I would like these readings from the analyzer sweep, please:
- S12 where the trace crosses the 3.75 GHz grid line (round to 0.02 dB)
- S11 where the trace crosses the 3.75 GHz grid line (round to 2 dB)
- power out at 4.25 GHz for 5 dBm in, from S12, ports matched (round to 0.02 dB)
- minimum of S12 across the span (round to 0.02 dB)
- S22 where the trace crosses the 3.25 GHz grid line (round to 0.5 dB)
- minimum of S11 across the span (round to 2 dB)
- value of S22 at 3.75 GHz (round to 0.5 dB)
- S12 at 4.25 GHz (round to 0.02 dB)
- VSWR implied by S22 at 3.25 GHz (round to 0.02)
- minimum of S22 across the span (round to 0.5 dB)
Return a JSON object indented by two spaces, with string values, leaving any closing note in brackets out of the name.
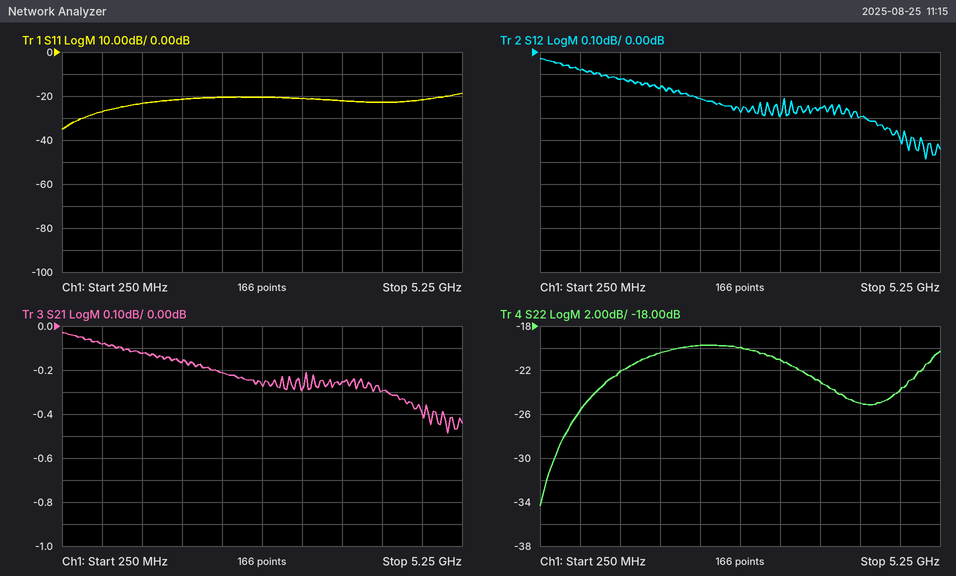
{
  "S12 where the trace crosses the 3.75 GHz grid line": "-0.26 dB",
  "S11 where the trace crosses the 3.75 GHz grid line": "-22 dB",
  "power out at 4.25 GHz for 5 dBm in, from S12, ports matched": "4.70 dBm",
  "minimum of S12 across the span": "-0.48 dB",
  "S22 where the trace crosses the 3.25 GHz grid line": "-21.0 dB",
  "minimum of S11 across the span": "-36 dB",
  "value of S22 at 3.75 GHz": "-23.0 dB",
  "S12 at 4.25 GHz": "-0.30 dB",
  "VSWR implied by S22 at 3.25 GHz": "1.20",
  "minimum of S22 across the span": "-34.5 dB"
}
